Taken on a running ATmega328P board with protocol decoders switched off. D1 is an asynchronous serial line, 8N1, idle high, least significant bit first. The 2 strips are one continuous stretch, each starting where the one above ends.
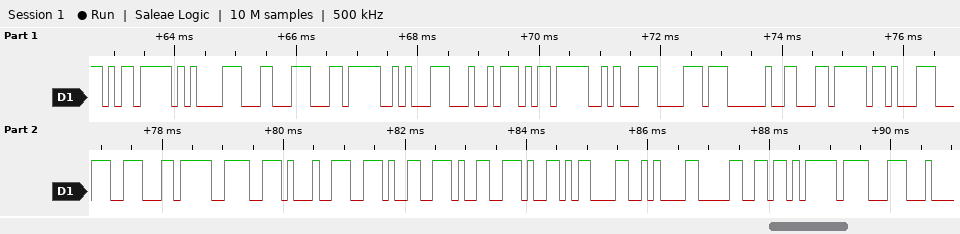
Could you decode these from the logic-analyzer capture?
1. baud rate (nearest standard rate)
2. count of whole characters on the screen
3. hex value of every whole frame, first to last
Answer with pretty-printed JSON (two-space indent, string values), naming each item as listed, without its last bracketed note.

{
  "baud rate": "9600 baud",
  "count of whole characters on the screen": "24",
  "hex value of every whole frame, first to last": "0xED 0x85 0x8C 0xEC 0x8A 0xA4 0xED 0x8A 0xB8 0x20 0xEC 0x8B 0x9C 0xEC 0x9E 0x91 0x2E 0x2E 0x2E 0x0D 0x0A 0x30 0xEB 0x8F"
}
